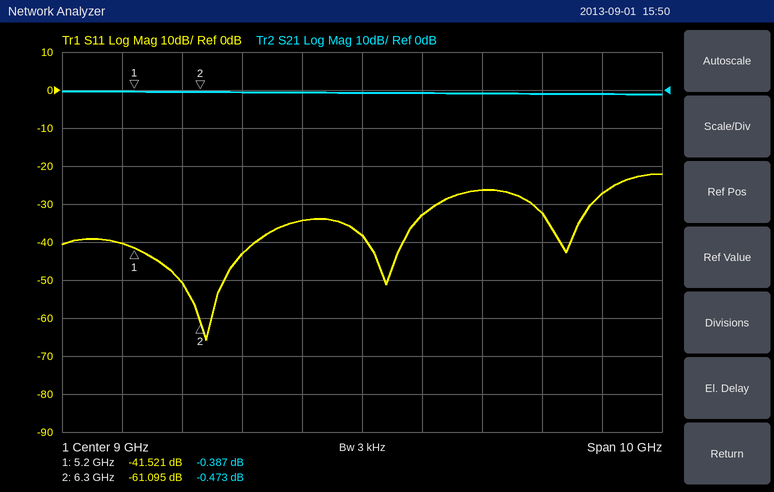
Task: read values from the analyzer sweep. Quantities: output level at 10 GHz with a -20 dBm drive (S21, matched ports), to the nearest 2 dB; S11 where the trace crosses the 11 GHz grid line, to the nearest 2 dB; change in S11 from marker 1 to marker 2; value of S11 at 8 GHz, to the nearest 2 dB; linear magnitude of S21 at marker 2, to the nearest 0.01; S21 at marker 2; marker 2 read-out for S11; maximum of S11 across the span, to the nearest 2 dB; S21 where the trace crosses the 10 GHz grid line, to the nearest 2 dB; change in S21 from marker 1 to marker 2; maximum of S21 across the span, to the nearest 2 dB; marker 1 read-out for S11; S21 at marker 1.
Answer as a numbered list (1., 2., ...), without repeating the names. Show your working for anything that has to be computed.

1. -20 dBm + (0 dB) = -20 dBm
2. -26 dB
3. -61.095 − (-41.521) = -19.574 dB
4. -34 dB
5. 10^(-0.473/20) ≈ 0.95
6. -0.473 dB
7. -61.095 dB
8. -22 dB
9. 0 dB
10. -0.473 − (-0.387) = -0.086 dB
11. 0 dB
12. -41.521 dB
13. -0.387 dB
